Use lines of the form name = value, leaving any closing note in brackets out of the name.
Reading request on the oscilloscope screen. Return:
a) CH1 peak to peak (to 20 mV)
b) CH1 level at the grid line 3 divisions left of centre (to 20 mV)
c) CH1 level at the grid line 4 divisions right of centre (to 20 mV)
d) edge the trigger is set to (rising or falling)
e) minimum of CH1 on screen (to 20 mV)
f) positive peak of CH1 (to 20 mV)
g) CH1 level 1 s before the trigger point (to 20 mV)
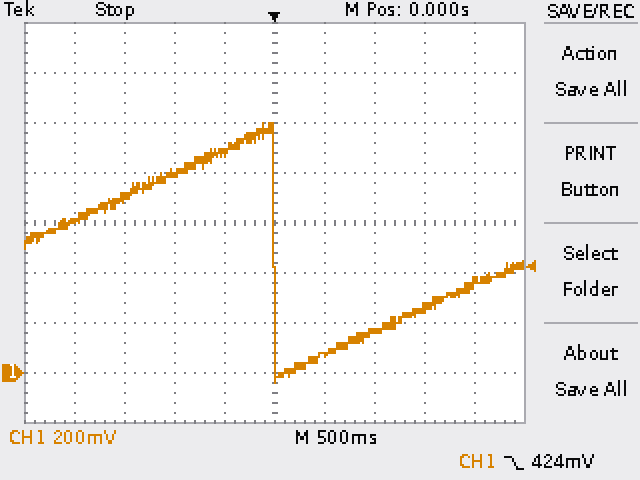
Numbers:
CH1 peak to peak = 1.04 V
CH1 level at the grid line 3 divisions left of centre = 700 mV
CH1 level at the grid line 4 divisions right of centre = 360 mV
edge the trigger is set to = falling
minimum of CH1 on screen = -40 mV
positive peak of CH1 = 1.00 V
CH1 level 1 s before the trigger point = 800 mV
